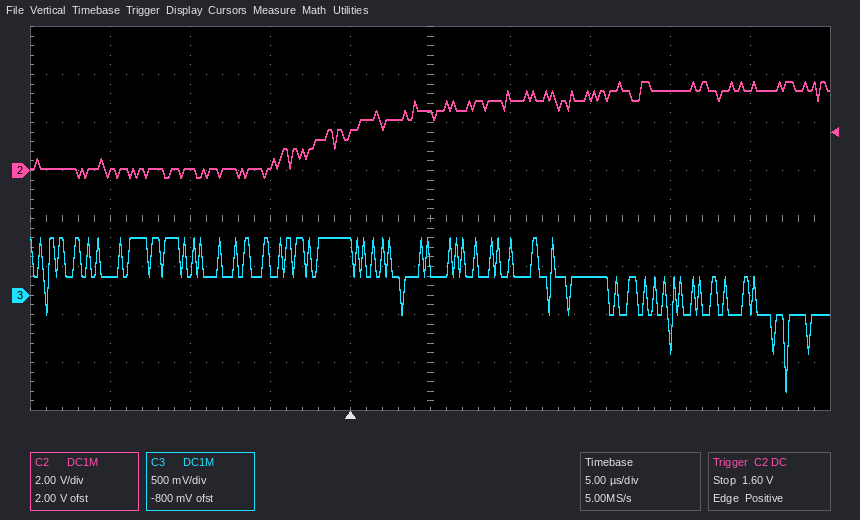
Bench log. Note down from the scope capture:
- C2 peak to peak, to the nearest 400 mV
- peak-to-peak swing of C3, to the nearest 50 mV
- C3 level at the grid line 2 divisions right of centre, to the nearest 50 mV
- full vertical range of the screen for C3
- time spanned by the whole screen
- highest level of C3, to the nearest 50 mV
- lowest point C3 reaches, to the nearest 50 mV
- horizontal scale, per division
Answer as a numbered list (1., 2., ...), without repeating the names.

1. 4.0 V
2. 1.60 V
3. 200 mV
4. 4 V
5. 50 µs
6. 600 mV
7. -1.00 V
8. 5 µs
